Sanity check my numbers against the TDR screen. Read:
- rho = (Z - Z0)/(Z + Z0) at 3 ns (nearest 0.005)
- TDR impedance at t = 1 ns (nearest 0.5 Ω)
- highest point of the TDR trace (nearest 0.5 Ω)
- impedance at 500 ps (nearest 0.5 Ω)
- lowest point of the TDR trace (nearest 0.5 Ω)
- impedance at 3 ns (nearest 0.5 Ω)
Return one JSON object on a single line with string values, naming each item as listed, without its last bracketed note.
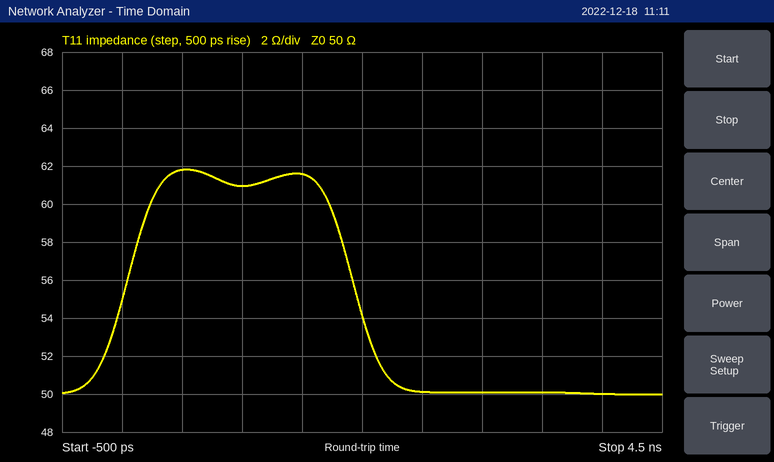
{"rho = (Z - Z0)/(Z + Z0) at 3 ns": "0.000", "TDR impedance at t = 1 ns": "61.0 Ω", "highest point of the TDR trace": "62.0 Ω", "impedance at 500 ps": "62.0 Ω", "lowest point of the TDR trace": "50.0 Ω", "impedance at 3 ns": "50.0 Ω"}
